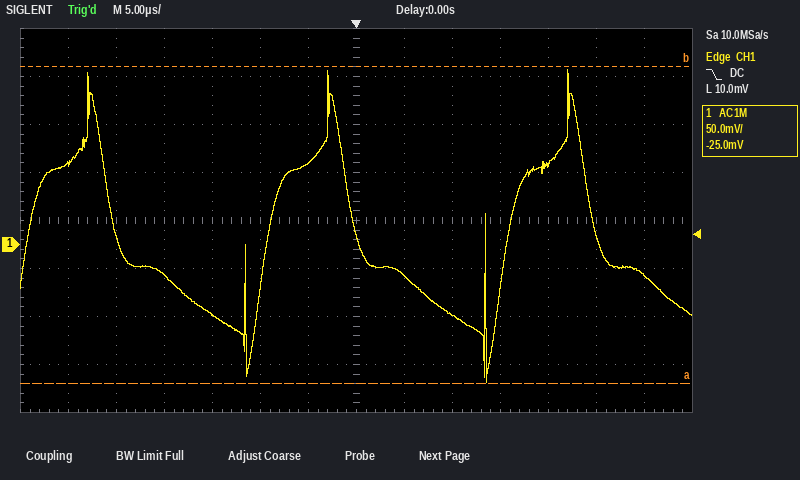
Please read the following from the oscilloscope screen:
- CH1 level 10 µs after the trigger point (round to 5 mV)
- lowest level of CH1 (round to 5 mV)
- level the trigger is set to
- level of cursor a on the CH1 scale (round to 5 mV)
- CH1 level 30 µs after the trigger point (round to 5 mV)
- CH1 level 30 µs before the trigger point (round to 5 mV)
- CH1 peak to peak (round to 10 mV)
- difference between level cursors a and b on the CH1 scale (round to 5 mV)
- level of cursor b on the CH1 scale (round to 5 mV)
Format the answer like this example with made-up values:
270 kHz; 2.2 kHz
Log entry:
-75 mV; -145 mV; 10.0 mV; -145 mV; -30 mV; 85 mV; 330 mV; 330 mV; 185 mV
